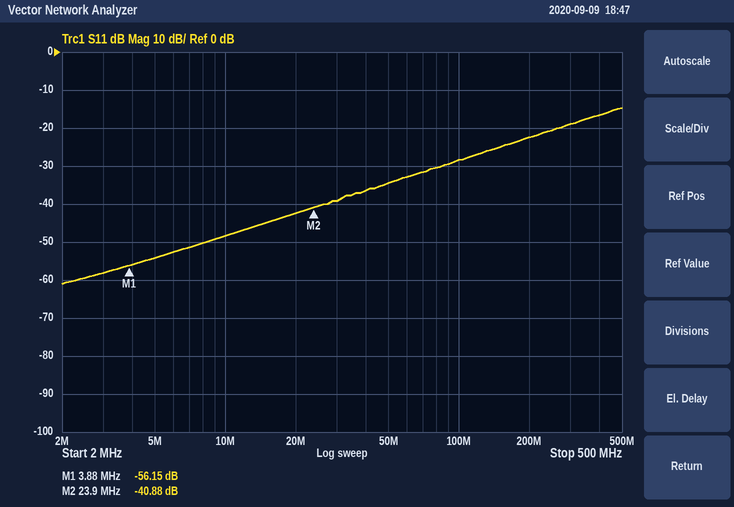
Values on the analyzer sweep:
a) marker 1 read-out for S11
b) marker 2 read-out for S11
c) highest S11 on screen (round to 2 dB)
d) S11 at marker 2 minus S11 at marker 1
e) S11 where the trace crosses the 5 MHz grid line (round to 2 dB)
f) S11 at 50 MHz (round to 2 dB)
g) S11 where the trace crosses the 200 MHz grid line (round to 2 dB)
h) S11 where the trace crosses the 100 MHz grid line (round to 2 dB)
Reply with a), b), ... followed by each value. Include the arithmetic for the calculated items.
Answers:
a) -56.15 dB
b) -40.88 dB
c) -14 dB
d) -40.88 − (-56.15) = 15.27 dB
e) -54 dB
f) -34 dB
g) -22 dB
h) -28 dB
